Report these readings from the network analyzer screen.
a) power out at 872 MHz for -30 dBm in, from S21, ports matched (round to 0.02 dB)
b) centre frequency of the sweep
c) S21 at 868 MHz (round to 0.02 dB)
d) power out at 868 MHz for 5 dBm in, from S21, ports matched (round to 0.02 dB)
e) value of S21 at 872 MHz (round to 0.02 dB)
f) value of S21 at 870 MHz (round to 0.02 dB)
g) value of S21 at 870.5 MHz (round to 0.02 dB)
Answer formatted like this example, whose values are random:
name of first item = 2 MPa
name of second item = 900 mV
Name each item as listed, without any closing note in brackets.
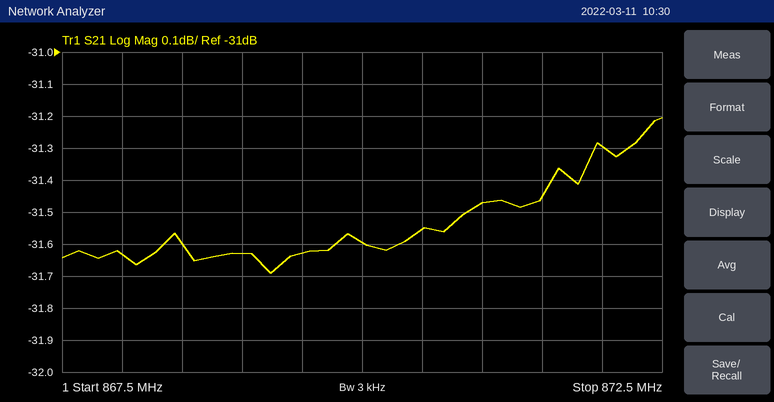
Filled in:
power out at 872 MHz for -30 dBm in, from S21, ports matched = -61.30 dBm
centre frequency of the sweep = 870 MHz
S21 at 868 MHz = -31.64 dB
power out at 868 MHz for 5 dBm in, from S21, ports matched = -26.64 dBm
value of S21 at 872 MHz = -31.30 dB
value of S21 at 870 MHz = -31.60 dB
value of S21 at 870.5 MHz = -31.56 dB
